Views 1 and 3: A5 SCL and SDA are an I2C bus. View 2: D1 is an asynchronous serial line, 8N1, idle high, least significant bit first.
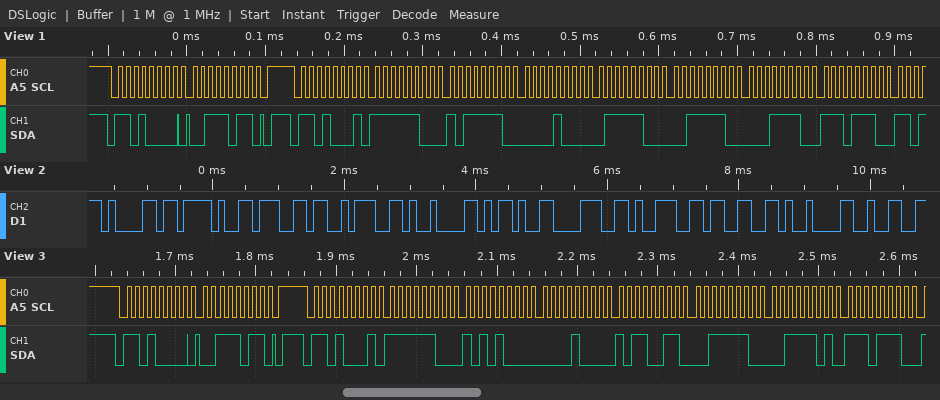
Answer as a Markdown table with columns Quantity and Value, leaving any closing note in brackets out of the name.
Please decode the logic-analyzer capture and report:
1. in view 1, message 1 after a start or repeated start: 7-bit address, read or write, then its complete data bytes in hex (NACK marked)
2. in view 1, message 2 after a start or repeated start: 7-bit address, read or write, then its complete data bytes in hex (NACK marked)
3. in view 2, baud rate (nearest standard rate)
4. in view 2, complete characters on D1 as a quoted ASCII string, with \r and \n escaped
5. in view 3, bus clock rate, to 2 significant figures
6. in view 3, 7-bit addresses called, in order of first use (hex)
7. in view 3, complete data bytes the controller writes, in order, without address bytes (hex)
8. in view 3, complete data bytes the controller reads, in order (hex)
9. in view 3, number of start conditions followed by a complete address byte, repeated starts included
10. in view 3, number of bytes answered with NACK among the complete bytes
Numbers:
| Quantity | Value |
|---|---|
| in view 1, message 1 after a start or repeated start: 7-bit address, read or write, then its complete data bytes in hex | 0x68 write: 3B |
| in view 1, message 2 after a start or repeated start: 7-bit address, read or write, then its complete data bytes in hex | 0x68 read: FC BE 08 7C 3E 1E EE |
| in view 2, baud rate | 9600 baud |
| in view 2, complete characters on D1 as a quoted ASCII string, with \r and \n escaped | "a/g:\t-893\t2" |
| in view 3, bus clock rate, to 2 significant figures | 100 kHz |
| in view 3, 7-bit addresses called, in order of first use | 0x68 |
| in view 3, complete data bytes the controller writes, in order, without address bytes | 3B |
| in view 3, complete data bytes the controller reads, in order | FC A8 08 B3 3E 3D EE |
| in view 3, number of start conditions followed by a complete address byte, repeated starts included | 2 |
| in view 3, number of bytes answered with NACK among the complete bytes | 0 |
